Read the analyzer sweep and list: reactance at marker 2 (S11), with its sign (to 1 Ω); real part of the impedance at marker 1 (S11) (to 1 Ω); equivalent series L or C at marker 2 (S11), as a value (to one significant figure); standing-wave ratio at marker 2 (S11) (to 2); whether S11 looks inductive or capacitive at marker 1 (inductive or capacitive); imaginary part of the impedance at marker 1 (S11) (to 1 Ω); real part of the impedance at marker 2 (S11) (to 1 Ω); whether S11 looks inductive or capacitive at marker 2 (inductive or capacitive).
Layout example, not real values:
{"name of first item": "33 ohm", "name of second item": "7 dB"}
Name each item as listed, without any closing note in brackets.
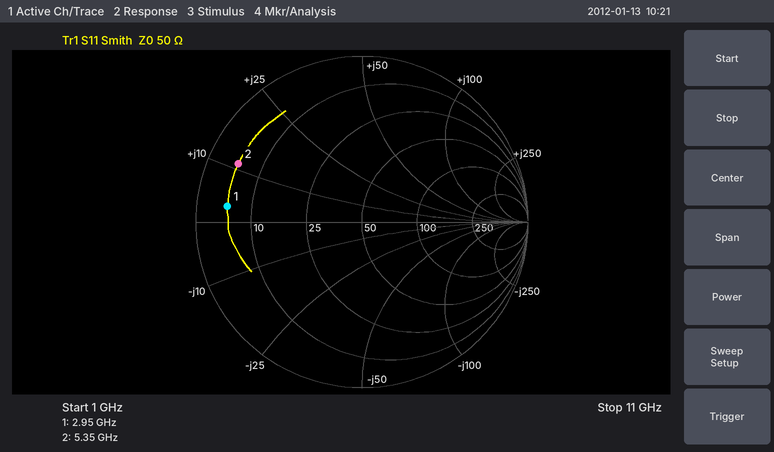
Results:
{"reactance at marker 2 (S11), with its sign": "+11 Ω", "real part of the impedance at marker 1 (S11)": "5 Ω", "equivalent series L or C at marker 2 (S11), as a value": "300 pH", "standing-wave ratio at marker 2 (S11)": "10", "whether S11 looks inductive or capacitive at marker 1": "inductive", "imaginary part of the impedance at marker 1 (S11)": "+3 Ω", "real part of the impedance at marker 2 (S11)": "5 Ω", "whether S11 looks inductive or capacitive at marker 2": "inductive"}
